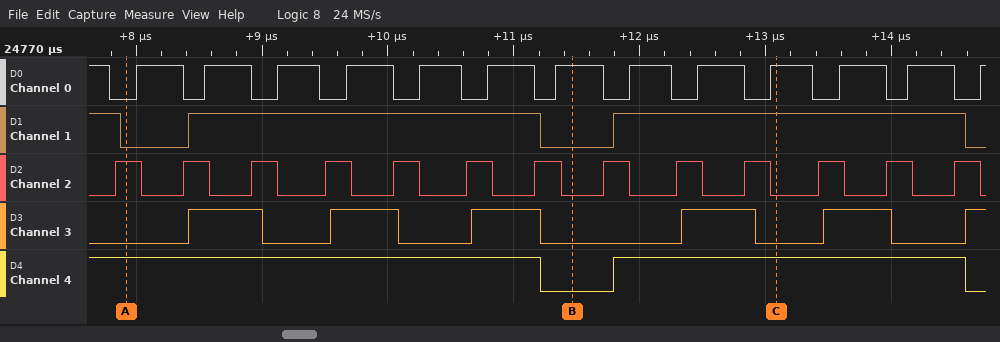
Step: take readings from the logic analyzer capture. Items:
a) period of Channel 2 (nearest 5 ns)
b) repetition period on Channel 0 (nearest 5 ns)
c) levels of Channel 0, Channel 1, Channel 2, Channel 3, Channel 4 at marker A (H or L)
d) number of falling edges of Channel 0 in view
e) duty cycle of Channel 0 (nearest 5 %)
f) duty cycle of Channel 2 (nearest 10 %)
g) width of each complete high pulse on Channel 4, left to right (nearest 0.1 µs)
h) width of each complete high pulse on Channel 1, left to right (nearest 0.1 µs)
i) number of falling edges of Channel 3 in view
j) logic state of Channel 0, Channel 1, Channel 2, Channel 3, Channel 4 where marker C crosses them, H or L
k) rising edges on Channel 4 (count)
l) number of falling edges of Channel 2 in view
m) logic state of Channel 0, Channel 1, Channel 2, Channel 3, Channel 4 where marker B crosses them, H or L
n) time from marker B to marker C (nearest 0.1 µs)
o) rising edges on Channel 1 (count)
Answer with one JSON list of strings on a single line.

["555 ns", "560 ns", "Channel 0=L, Channel 1=L, Channel 2=H, Channel 3=L, Channel 4=H", "13", "65 %", "40 %", "2.8 µs", "2.8 µs, 2.8 µs", "5", "Channel 0=H, Channel 1=H, Channel 2=L, Channel 3=L, Channel 4=H", "1", "13", "Channel 0=H, Channel 1=L, Channel 2=L, Channel 3=L, Channel 4=L", "1.6 µs", "2"]
